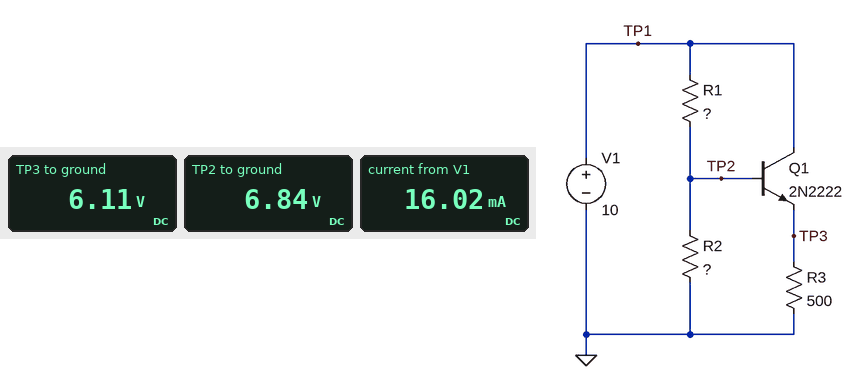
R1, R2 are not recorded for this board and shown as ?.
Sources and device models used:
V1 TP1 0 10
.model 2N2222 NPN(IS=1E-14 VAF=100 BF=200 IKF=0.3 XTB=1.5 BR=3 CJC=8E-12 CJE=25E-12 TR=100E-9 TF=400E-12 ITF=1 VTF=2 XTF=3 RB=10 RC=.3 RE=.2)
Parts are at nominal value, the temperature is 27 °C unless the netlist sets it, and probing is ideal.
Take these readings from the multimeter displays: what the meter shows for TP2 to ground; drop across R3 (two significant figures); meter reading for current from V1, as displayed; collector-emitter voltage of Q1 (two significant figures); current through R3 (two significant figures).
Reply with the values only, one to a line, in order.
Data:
6.84 V
6.1 V
16.02 mA
3.9 V
12 mA
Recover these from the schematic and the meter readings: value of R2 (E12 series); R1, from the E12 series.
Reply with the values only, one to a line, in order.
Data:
1.8 kΩ
820 Ω
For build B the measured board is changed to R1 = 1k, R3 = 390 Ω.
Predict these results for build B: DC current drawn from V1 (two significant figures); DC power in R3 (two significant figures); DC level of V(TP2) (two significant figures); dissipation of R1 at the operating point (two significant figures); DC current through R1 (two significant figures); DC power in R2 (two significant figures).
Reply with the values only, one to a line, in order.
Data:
18 mA
82 mW
6.4 V
13 mW
3.6 mA
23 mW
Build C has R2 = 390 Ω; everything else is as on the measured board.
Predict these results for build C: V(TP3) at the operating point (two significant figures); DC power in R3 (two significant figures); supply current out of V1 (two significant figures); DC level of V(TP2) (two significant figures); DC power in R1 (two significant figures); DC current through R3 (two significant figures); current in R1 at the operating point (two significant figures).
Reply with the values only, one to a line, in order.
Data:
2.5 V
13 mW
13 mA
3.2 V
56 mW
5.0 mA
8.3 mA
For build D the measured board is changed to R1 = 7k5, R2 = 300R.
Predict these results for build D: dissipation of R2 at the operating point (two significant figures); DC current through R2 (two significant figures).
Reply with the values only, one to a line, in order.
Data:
490 µW
1.3 mA
